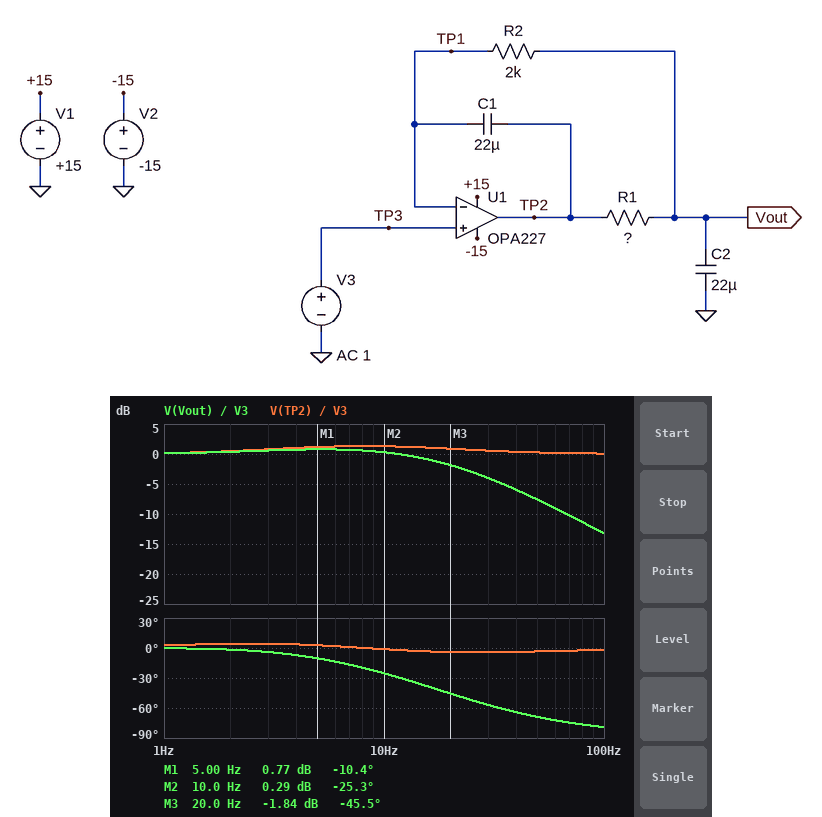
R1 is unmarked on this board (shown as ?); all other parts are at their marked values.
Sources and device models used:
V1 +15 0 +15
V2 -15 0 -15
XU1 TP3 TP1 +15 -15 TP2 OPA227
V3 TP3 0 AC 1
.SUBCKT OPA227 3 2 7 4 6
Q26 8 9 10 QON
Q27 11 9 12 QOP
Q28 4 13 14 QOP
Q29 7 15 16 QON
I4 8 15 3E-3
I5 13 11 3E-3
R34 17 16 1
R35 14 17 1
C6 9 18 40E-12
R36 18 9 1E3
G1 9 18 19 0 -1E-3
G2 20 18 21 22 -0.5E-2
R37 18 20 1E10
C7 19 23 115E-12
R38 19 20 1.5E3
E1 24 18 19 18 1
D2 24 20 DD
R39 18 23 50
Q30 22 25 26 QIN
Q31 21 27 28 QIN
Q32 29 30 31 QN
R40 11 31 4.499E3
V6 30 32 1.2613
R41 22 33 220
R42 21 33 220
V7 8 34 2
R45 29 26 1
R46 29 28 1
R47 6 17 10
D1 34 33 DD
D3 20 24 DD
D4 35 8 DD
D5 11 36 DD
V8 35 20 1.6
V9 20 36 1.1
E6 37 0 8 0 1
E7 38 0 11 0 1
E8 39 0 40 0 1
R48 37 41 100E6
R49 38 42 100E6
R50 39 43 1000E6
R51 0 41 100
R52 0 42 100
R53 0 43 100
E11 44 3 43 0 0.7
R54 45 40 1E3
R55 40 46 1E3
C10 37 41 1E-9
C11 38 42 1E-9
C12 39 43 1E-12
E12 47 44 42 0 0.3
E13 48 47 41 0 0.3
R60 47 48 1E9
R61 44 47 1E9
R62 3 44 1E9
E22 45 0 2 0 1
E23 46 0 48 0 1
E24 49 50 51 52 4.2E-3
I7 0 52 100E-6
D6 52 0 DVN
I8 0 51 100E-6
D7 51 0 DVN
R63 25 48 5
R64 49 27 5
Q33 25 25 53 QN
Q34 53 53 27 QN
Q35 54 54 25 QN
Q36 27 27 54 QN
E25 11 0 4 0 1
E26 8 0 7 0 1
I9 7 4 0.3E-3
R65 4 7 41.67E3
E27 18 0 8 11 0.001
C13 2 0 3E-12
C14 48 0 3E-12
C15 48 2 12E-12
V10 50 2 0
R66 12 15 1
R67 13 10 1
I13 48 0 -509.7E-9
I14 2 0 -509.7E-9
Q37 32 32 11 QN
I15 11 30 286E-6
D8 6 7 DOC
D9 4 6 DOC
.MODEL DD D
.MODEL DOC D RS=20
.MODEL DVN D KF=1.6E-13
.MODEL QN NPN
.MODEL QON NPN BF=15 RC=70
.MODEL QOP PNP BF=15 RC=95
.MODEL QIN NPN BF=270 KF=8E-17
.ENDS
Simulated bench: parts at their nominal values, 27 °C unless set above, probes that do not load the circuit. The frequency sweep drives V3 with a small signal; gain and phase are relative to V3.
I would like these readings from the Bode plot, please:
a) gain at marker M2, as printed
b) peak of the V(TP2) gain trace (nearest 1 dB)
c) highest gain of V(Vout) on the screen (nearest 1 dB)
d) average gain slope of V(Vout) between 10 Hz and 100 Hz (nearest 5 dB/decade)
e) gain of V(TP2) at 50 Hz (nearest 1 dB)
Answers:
0.29 dB
1 dB
1 dB
-15 dB/decade
0 dB
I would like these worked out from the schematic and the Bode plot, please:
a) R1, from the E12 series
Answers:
390 Ω
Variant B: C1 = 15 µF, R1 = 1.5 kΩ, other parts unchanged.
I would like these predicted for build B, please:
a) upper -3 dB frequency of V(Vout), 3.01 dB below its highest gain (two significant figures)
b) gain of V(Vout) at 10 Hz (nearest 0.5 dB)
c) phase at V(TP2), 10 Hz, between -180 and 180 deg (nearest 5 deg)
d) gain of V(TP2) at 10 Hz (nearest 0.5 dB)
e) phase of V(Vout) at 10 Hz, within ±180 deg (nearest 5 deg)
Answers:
9.0 Hz
-2.0 dB
-15 deg
3.0 dB
-60 deg
